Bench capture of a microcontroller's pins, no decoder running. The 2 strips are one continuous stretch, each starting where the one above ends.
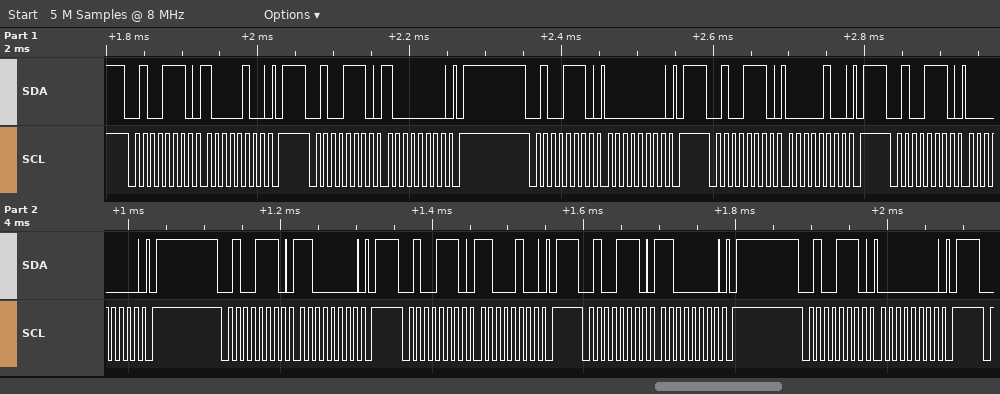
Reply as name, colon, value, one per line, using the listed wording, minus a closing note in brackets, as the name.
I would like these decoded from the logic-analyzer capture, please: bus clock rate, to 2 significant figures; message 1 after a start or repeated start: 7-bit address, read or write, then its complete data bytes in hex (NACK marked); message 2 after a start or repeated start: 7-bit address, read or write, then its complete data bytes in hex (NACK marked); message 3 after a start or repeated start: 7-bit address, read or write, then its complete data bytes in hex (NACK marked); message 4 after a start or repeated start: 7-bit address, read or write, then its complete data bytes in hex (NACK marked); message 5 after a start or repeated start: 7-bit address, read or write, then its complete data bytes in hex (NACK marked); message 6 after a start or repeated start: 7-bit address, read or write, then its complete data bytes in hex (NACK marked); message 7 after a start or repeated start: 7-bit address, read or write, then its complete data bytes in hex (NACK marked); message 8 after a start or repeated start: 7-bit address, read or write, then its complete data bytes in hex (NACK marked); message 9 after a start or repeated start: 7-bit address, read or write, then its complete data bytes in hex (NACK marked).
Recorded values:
bus clock rate, to 2 significant figures: 100 kHz
message 1 after a start or repeated start: 7-bit address, read or write, then its complete data bytes in hex: 0x27 write: 84
message 2 after a start or repeated start: 7-bit address, read or write, then its complete data bytes in hex: 0x27 write: 80
message 3 after a start or repeated start: 7-bit address, read or write, then its complete data bytes in hex: 0x27 write: 00
message 4 after a start or repeated start: 7-bit address, read or write, then its complete data bytes in hex: 0x27 write: 04
message 5 after a start or repeated start: 7-bit address, read or write, then its complete data bytes in hex: 0x27 write: 00
message 6 after a start or repeated start: 7-bit address, read or write, then its complete data bytes in hex: 0x27 write: C0
message 7 after a start or repeated start: 7-bit address, read or write, then its complete data bytes in hex: 0x27 write: C4
message 8 after a start or repeated start: 7-bit address, read or write, then its complete data bytes in hex: 0x27 write: C0
message 9 after a start or repeated start: 7-bit address, read or write, then its complete data bytes in hex: 0x27 write: 00
